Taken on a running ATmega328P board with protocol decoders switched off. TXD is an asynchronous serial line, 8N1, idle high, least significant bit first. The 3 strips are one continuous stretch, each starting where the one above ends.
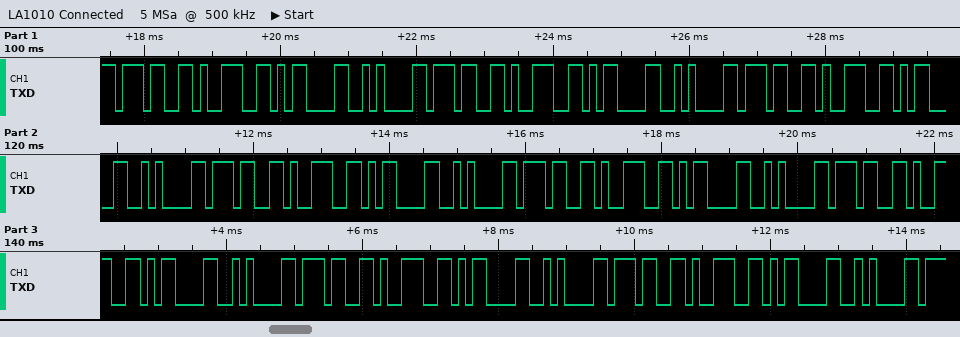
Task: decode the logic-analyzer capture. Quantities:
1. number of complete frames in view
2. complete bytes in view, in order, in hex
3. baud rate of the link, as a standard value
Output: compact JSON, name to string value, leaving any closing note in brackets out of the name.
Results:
{"number of complete frames in view": "32", "complete bytes in view, in order, in hex": "37 39 0D 0A 37 39 0D 0A 37 39 0D 0A 37 39 0D 0A 37 39 0D 0A 37 39 0D 0A 37 39 0D 0A 37 39 0D 0A", "baud rate of the link, as a standard value": "9600 baud"}
